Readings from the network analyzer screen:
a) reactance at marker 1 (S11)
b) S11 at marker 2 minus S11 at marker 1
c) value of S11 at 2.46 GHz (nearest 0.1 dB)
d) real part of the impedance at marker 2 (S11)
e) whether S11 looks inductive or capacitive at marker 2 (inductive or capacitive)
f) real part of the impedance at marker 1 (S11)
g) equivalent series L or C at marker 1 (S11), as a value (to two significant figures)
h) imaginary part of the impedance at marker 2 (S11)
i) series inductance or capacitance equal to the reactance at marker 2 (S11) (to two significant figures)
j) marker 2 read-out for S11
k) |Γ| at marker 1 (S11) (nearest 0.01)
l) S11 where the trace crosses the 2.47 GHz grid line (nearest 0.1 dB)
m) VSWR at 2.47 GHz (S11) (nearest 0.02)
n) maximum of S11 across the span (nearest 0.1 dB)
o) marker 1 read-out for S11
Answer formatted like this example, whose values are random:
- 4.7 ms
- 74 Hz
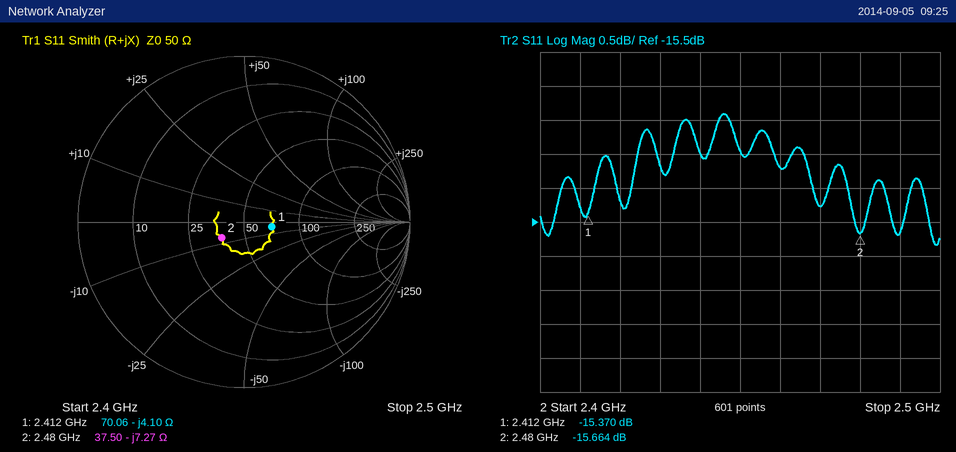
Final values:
- -4.10 Ω
- -0.294 dB
- -14.7 dB
- 37.50 Ω
- capacitive
- 70.06 Ω
- 16 pF
- -7.27 Ω
- 8.8 pF
- -15.664 dB
- 0.17
- -15.3 dB
- 1.42
- -13.9 dB
- -15.370 dB
